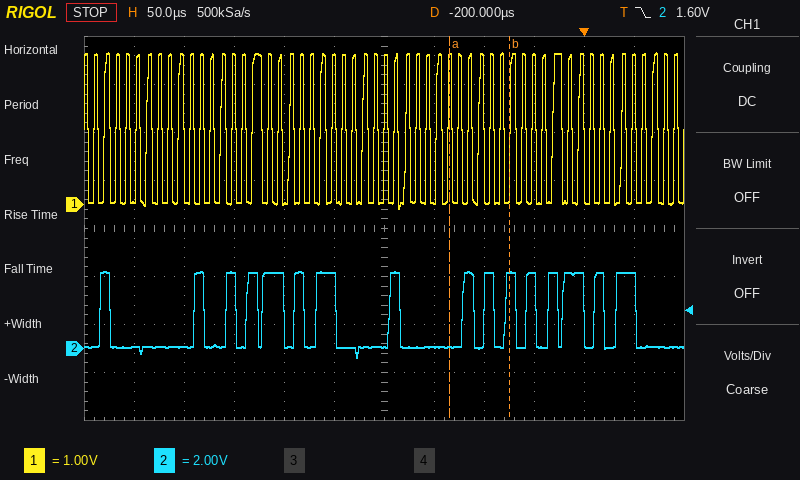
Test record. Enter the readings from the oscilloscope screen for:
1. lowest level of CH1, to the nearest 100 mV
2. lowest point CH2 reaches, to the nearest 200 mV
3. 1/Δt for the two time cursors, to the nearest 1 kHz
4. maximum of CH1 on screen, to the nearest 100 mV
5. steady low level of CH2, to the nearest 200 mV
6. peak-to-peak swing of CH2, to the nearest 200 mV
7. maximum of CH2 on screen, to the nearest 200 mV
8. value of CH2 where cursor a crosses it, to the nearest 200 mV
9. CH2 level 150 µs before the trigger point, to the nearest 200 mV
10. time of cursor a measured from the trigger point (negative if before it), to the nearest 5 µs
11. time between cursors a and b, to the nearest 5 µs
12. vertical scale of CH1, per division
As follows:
-100 mV
-400 mV
17 kHz
3.2 V
0.0 V
3.6 V
3.2 V
0.0 V
0.0 V
-135 µs
60 µs
1 V
